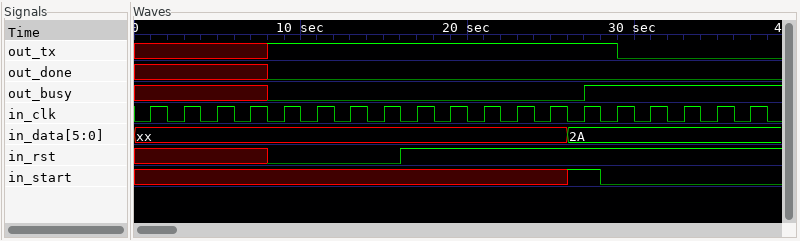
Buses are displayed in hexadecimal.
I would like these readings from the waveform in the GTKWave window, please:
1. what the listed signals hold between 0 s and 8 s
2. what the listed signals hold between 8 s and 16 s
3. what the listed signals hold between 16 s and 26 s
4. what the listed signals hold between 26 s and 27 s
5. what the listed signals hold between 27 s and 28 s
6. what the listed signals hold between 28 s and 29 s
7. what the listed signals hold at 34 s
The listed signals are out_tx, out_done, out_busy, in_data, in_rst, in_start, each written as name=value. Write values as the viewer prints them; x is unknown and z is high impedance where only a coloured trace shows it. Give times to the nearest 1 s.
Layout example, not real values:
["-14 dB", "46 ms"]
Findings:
["out_tx=x, out_done=x, out_busy=x, in_data=xx, in_rst=x, in_start=x", "out_tx=1, out_done=0, out_busy=0, in_data=xx, in_rst=0, in_start=x", "out_tx=1, out_done=0, out_busy=0, in_data=xx, in_rst=1, in_start=x", "out_tx=1, out_done=0, out_busy=0, in_data=2A, in_rst=1, in_start=1", "out_tx=1, out_done=0, out_busy=1, in_data=2A, in_rst=1, in_start=1", "out_tx=1, out_done=0, out_busy=1, in_data=2A, in_rst=1, in_start=0", "out_tx=0, out_done=0, out_busy=1, in_data=2A, in_rst=1, in_start=0"]
